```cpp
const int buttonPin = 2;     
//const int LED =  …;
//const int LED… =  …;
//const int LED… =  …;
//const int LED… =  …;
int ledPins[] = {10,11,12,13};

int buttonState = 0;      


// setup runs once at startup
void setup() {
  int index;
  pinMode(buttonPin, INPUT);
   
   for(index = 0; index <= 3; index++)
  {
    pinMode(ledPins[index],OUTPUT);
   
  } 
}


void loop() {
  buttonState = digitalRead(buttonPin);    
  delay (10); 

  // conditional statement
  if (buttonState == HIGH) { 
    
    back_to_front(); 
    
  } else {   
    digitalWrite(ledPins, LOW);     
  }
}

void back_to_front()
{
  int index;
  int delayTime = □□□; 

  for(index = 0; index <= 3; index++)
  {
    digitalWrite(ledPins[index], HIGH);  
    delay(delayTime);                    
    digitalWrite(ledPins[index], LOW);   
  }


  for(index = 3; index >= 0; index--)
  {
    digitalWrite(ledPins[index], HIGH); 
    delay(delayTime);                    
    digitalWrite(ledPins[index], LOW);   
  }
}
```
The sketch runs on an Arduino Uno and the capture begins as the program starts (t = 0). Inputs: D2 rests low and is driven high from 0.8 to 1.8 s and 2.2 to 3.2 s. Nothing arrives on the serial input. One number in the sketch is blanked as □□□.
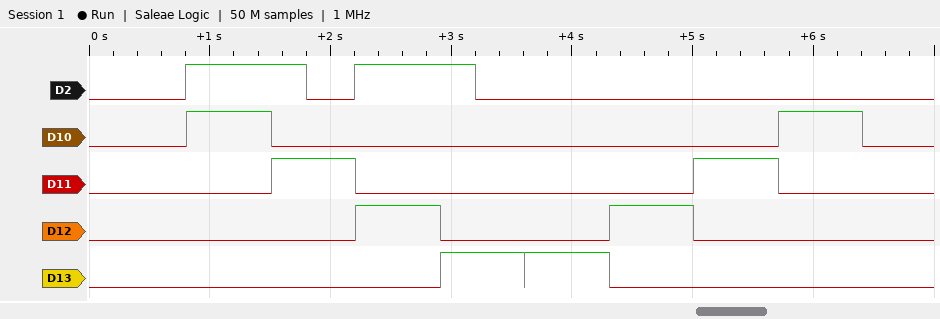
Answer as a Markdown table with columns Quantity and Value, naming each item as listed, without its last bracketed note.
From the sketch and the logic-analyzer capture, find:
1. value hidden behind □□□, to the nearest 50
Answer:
| Quantity | Value |
|---|---|
| value hidden behind □□□, to the nearest 50 | 700 |
